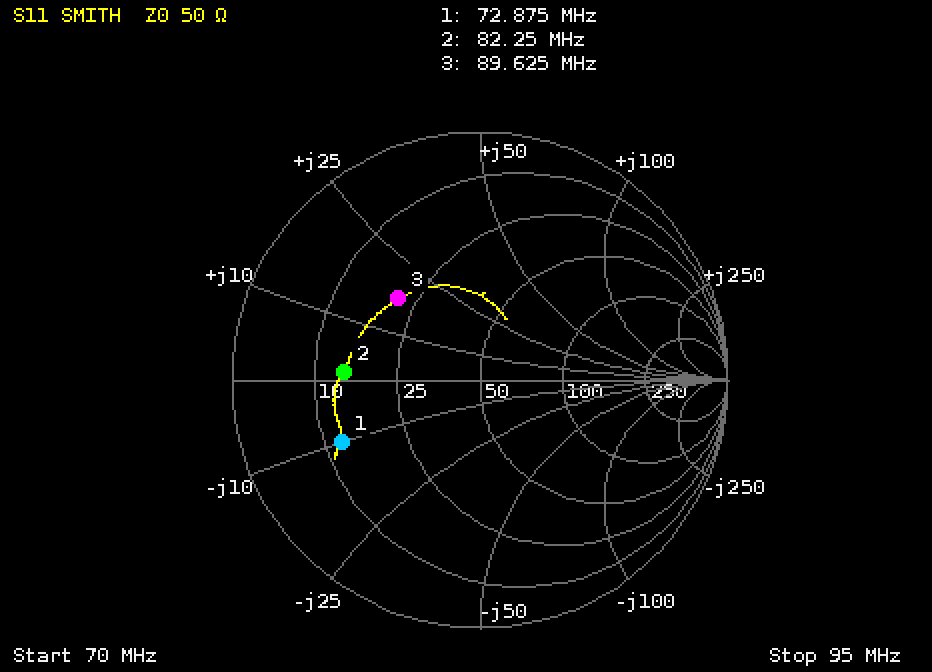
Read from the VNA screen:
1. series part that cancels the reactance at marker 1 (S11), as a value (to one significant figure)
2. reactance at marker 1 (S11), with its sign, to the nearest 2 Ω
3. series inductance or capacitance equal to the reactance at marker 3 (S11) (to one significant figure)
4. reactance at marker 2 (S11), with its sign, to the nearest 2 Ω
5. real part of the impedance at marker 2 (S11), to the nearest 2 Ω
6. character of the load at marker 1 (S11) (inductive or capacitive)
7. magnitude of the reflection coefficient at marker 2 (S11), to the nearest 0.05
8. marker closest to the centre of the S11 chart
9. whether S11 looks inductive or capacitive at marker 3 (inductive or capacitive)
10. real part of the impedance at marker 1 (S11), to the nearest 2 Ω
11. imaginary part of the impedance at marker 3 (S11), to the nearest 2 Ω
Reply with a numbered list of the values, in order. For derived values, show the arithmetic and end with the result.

1. L = 10 Ω/(2π × 72.875 MHz) ≈ 21.8 nH, so 20 nH to one significant figure
2. -10 Ω
3. L = 18 Ω/(2π × 89.625 MHz) ≈ 32.0 nH, so 30 nH to one significant figure
4. +2 Ω
5. 14 Ω
6. capacitive
7. 0.55
8. marker 3
9. inductive
10. 12 Ω
11. +18 Ω
